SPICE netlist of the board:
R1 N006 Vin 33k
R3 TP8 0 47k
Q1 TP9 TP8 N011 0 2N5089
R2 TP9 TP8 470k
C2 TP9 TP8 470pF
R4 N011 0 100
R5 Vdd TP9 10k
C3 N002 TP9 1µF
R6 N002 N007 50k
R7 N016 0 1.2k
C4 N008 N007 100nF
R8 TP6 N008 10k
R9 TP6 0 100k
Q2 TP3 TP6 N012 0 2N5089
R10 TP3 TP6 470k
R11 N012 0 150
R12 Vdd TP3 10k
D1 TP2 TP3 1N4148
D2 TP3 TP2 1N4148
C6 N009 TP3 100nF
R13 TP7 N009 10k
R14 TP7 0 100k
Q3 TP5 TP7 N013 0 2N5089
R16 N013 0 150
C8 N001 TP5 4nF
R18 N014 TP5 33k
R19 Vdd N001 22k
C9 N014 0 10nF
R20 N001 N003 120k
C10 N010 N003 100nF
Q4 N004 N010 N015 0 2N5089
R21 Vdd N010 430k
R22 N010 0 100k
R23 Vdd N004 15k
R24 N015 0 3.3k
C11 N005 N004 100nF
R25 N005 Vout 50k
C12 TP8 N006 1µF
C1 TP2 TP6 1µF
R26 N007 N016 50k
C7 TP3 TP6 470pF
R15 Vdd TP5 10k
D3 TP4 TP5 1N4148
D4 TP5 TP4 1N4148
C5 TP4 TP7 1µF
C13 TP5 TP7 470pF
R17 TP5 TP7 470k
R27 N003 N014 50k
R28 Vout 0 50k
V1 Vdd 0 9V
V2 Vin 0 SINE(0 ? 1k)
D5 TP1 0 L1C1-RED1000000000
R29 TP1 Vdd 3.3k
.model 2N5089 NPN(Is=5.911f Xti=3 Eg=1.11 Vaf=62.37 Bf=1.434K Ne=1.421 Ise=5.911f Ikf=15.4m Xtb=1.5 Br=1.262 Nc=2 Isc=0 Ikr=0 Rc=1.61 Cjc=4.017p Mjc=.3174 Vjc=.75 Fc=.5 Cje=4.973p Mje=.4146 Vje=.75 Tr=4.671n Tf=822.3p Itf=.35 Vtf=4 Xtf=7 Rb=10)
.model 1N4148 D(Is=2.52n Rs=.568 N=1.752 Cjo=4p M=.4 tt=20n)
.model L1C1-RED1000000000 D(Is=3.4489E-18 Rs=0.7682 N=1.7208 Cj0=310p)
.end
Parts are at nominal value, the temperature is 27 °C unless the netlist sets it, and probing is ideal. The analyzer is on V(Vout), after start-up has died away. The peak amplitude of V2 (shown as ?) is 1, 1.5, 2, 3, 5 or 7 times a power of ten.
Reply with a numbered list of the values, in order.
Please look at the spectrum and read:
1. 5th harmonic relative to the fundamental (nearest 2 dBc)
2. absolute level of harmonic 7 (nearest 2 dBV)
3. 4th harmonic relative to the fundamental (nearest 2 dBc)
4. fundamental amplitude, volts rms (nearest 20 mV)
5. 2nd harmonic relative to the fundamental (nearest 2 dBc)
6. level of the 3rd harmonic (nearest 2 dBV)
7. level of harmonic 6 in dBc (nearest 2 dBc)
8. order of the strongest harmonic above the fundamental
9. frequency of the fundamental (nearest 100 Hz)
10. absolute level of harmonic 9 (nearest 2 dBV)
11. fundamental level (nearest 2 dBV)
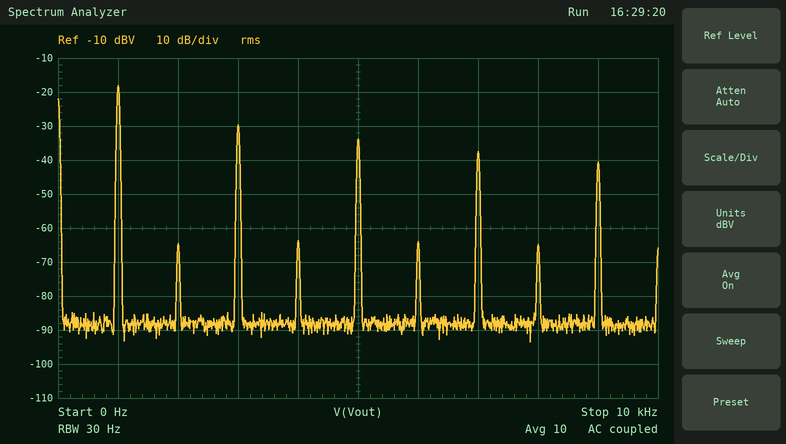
1. -16 dBc
2. -38 dBV
3. -46 dBc
4. 120 mV
5. -46 dBc
6. -30 dBV
7. -46 dBc
8. 3
9. 1.0 kHz
10. -40 dBV
11. -18 dBV
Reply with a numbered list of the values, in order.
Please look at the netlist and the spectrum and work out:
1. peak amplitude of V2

1. 70 mV
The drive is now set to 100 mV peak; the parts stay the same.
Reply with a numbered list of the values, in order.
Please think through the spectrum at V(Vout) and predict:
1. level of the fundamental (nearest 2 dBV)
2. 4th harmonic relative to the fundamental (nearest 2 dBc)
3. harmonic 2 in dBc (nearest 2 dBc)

1. -18 dBV
2. -42 dBc
3. -42 dBc
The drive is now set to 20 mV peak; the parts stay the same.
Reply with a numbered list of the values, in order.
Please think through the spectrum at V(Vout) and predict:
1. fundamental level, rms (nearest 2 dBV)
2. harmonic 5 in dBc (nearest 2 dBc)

1. -18 dBV
2. -18 dBc
